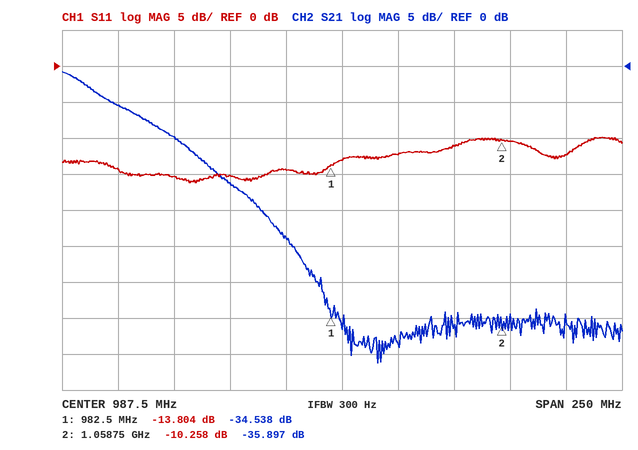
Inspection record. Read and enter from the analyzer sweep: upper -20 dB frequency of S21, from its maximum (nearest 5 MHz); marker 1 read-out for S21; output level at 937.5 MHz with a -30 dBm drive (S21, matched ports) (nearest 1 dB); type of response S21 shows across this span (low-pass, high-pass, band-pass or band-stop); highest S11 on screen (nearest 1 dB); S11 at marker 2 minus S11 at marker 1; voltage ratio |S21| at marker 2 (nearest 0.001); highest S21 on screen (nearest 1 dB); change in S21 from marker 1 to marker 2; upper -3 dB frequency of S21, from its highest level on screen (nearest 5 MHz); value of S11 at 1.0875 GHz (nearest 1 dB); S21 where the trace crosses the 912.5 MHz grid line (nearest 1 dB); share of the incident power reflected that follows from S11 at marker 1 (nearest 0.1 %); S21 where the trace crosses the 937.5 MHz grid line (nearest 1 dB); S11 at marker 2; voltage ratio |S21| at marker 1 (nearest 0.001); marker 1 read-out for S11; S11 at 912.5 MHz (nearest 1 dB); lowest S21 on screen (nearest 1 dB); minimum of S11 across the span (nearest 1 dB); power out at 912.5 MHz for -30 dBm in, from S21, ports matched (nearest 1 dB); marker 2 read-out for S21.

955 MHz
-34.538 dB
-46 dBm
low-pass
-10 dB
3.546 dB
0.016
-1 dB
-1.359 dB
880 MHz
-12 dB
-10 dB
4.2 %
-16 dB
-10.258 dB
0.019
-13.804 dB
-15 dB
-41 dB
-16 dB
-40 dBm
-35.897 dB
